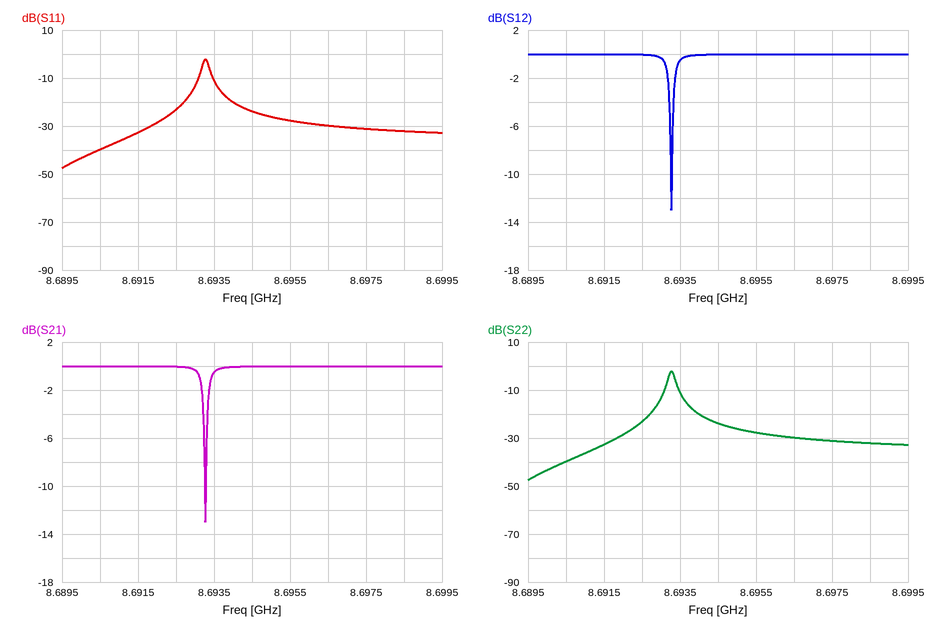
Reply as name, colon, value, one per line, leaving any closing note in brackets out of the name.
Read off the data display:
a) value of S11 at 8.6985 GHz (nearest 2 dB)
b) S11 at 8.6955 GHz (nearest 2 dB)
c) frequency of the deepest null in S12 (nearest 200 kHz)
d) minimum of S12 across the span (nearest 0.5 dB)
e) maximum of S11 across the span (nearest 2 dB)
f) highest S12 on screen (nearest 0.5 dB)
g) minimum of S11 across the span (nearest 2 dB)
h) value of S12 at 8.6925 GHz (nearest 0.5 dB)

value of S11 at 8.6985 GHz: -32 dB
S11 at 8.6955 GHz: -28 dB
frequency of the deepest null in S12: 8.6932 GHz
minimum of S12 across the span: -13.0 dB
maximum of S11 across the span: -2 dB
highest S12 on screen: 0.0 dB
minimum of S11 across the span: -48 dB
value of S12 at 8.6925 GHz: 0.0 dB
